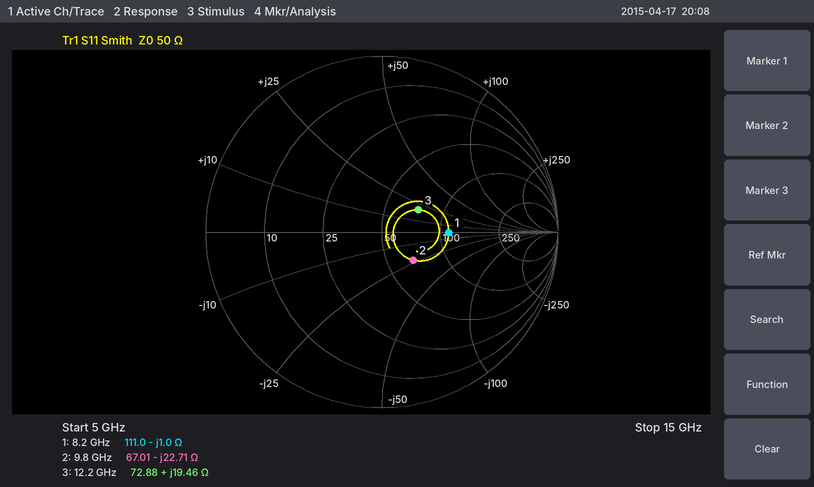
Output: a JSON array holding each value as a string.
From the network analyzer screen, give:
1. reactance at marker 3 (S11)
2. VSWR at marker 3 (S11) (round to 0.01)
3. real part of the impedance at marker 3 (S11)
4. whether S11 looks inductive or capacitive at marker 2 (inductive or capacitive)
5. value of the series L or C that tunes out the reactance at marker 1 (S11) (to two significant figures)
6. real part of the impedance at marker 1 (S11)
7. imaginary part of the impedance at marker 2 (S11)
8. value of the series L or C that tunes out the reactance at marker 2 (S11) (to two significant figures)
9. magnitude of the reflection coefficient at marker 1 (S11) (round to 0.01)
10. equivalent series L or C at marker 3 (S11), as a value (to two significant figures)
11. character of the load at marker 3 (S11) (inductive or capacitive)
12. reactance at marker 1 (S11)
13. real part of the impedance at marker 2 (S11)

["+19.46 Ω", "1.64", "72.88 Ω", "capacitive", "19 pH", "111.0 Ω", "-22.71 Ω", "370 pH", "0.38", "250 pH", "inductive", "-1.0 Ω", "67.01 Ω"]
